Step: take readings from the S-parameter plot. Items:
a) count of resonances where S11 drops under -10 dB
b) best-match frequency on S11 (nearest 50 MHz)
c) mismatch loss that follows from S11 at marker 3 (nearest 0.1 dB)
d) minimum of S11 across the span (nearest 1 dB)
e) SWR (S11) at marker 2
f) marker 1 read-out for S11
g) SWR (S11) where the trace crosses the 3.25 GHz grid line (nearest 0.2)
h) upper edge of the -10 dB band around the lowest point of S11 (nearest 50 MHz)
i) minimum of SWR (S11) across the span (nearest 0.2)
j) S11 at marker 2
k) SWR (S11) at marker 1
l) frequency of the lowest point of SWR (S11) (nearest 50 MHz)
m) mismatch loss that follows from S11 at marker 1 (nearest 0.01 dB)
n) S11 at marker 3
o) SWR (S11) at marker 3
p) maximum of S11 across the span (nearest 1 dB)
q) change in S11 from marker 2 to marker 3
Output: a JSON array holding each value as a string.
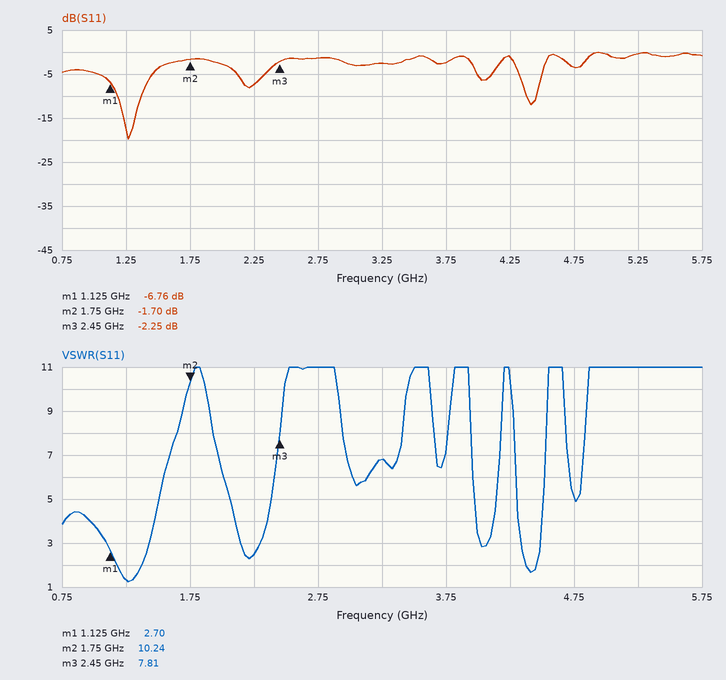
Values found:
["2", "1.25 GHz", "3.9 dB", "-20 dB", "10.24", "-6.76 dB", "6.8", "1.35 GHz", "1.2", "-1.70 dB", "2.70", "1.25 GHz", "1.03 dB", "-2.25 dB", "7.81", "0 dB", "-0.55 dB"]
